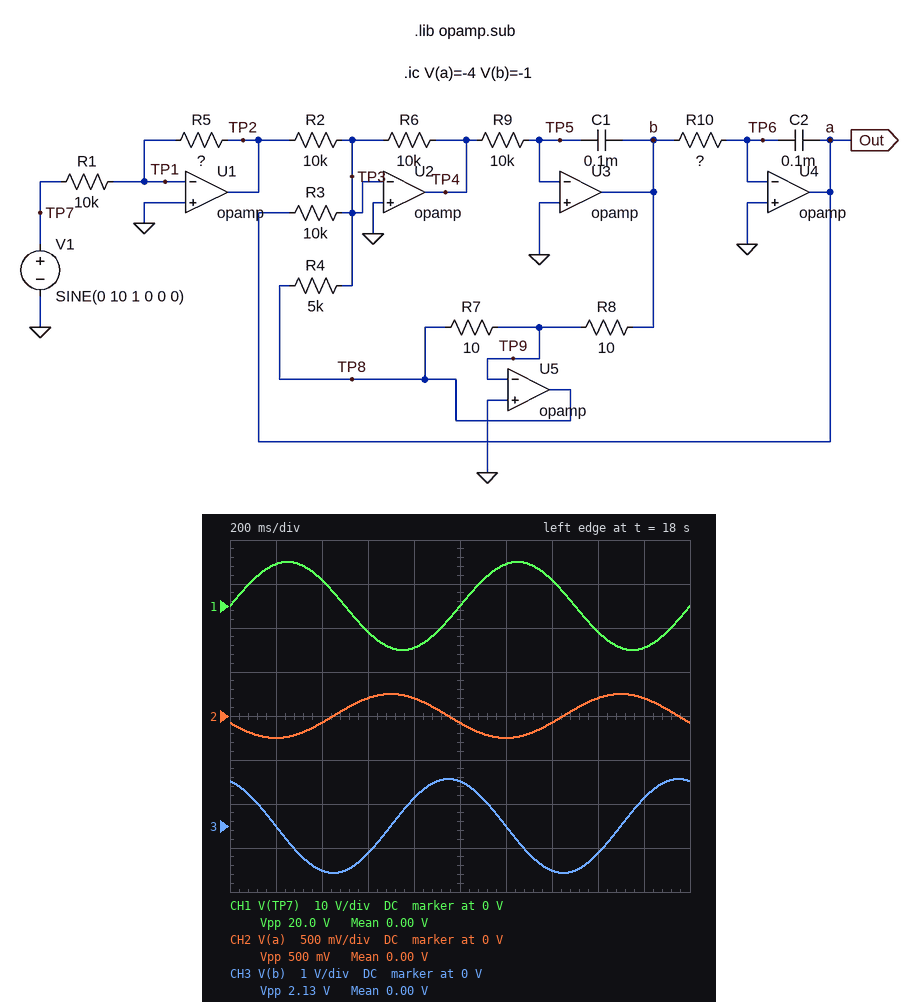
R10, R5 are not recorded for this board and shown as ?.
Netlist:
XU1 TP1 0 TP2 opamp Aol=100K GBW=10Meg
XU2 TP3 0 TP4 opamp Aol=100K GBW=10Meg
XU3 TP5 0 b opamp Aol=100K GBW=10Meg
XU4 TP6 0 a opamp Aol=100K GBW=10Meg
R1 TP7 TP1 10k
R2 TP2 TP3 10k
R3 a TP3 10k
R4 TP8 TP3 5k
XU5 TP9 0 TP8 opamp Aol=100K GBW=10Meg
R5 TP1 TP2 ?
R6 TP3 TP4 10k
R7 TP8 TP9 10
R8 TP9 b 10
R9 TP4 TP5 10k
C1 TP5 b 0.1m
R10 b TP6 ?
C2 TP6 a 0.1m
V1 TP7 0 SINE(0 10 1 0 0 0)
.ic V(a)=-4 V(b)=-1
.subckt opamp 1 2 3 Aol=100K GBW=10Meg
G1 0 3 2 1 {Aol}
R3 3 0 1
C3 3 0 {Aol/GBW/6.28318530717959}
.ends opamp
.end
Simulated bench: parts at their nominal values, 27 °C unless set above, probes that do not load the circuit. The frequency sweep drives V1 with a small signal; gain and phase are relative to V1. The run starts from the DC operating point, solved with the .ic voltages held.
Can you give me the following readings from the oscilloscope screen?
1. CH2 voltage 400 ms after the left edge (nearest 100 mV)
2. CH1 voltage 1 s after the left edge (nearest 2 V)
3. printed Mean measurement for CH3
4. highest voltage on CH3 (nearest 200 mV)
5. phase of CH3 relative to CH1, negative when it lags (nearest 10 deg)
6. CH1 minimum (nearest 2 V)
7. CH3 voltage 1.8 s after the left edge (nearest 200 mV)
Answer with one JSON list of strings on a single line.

["-100 mV", "0 V", "0.00 V", "1.0 V", "110 deg", "-10 V", "600 mV"]
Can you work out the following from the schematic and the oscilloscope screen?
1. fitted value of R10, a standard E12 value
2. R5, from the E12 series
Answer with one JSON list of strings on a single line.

["6.8 kΩ", "6.8 kΩ"]
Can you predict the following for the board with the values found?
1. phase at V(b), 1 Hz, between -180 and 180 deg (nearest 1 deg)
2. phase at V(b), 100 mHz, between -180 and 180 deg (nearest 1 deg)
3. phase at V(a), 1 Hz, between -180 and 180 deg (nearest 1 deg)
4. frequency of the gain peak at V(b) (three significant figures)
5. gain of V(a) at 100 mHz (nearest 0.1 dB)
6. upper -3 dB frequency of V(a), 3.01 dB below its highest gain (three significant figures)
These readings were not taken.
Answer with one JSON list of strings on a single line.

["108 deg", "-139 deg", "-162 deg", "193 mHz", "-4.4 dB", "162 mHz"]
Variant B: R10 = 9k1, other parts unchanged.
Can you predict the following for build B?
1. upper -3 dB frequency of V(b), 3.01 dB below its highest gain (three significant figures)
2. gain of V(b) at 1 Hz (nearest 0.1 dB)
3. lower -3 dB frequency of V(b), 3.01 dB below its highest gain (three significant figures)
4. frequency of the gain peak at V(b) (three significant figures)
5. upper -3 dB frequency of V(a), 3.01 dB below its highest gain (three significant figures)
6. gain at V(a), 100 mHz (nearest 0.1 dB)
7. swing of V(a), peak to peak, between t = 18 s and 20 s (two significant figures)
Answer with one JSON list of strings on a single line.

["390 mHz", "-19.5 dB", "71.4 mHz", "167 mHz", "115 mHz", "-5.7 dB", "370 mV"]
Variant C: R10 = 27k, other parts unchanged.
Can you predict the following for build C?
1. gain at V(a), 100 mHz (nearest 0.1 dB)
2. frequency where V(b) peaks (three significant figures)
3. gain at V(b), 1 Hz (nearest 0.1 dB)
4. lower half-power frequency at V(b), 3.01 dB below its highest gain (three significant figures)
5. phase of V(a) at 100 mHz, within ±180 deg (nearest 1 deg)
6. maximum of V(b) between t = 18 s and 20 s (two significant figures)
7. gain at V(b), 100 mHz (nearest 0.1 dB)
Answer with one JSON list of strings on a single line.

["-14.0 dB", "96.9 mHz", "-19.7 dB", "27.2 mHz", "-91 deg", "1.0 V", "-9.4 dB"]
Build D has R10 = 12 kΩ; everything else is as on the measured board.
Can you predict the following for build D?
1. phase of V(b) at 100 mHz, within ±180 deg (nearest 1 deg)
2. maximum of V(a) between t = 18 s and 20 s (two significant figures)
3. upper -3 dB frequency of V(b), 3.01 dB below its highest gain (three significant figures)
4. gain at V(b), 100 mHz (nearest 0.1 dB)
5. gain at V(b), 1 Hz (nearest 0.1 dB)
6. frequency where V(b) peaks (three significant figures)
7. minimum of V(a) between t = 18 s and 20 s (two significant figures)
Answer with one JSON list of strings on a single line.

["-161 deg", "140 mV", "375 mHz", "-9.9 dB", "-19.6 dB", "145 mHz", "-140 mV"]
